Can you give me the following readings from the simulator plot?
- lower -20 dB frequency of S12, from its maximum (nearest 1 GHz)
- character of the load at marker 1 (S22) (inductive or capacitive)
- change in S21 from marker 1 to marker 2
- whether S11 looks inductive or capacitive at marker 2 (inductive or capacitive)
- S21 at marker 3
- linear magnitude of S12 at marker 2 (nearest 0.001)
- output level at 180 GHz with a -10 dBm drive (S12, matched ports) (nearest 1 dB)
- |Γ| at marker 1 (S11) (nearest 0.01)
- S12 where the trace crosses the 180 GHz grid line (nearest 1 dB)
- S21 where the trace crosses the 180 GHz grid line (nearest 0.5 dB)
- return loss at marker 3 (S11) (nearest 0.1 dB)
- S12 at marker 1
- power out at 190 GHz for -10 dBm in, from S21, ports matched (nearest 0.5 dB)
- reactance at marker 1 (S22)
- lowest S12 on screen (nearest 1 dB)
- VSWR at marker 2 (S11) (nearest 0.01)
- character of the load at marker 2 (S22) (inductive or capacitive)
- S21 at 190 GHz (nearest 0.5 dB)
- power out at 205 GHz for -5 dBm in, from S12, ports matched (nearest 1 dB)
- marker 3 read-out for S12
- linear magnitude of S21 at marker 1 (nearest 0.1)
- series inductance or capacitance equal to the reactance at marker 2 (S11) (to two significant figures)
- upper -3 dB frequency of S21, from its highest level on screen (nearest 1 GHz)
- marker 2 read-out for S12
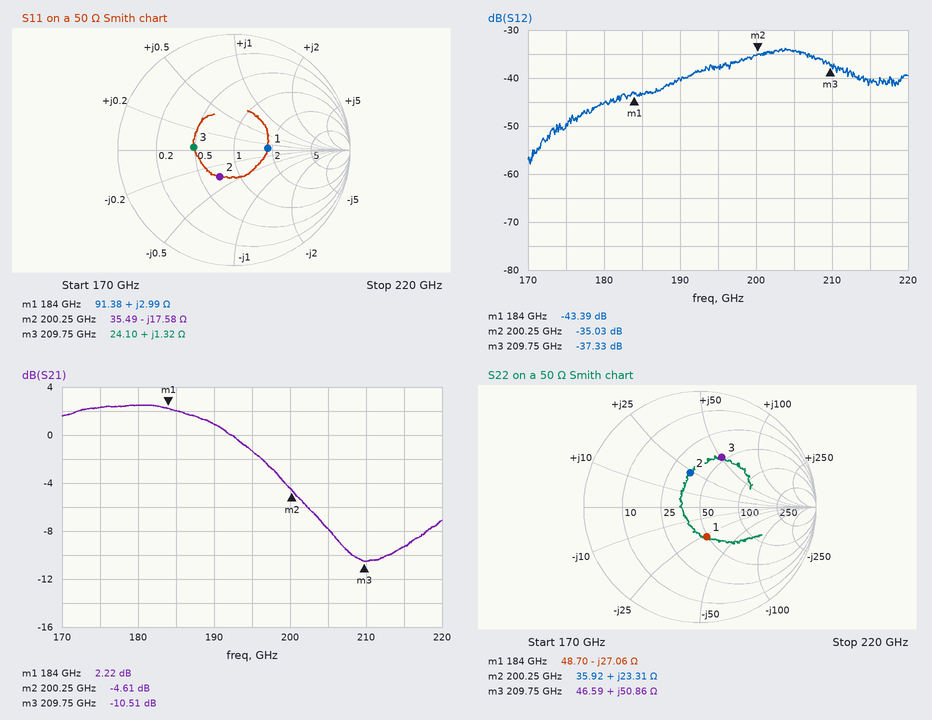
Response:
172 GHz
capacitive
-6.83 dB
capacitive
-10.51 dB
0.018
-55 dBm
0.29
-45 dB
2.5 dB
9.1 dB
-43.39 dB
-9.0 dBm
-27.06 Ω
-58 dB
1.71
inductive
1.0 dB
-39 dBm
-37.33 dB
1.3
45 fF
193 GHz
-35.03 dB
